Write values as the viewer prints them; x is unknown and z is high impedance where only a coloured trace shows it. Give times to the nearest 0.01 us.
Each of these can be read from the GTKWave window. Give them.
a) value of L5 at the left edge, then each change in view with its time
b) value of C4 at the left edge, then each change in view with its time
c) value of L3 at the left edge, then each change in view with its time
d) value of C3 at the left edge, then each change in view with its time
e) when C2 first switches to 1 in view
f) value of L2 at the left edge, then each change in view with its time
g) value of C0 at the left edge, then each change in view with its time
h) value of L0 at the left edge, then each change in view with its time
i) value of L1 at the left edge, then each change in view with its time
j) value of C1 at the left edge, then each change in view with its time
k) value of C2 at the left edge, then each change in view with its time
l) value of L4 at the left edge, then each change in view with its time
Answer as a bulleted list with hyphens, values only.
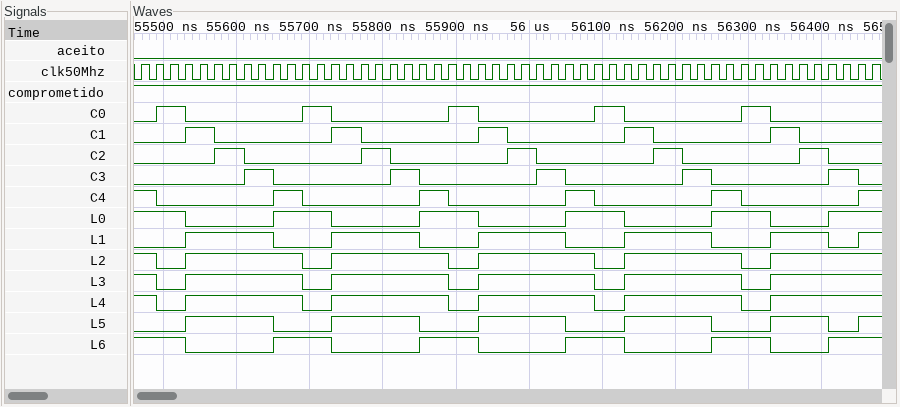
- 0, 1 at 55.53 us, 0 at 55.65 us, 1 at 55.73 us, 0 at 55.85 us, 1 at 55.93 us, 0 at 56.05 us, 1 at 56.13 us, 0 at 56.25 us, 1 at 56.33 us, 0 at 56.41 us, 1 at 56.45 us
- 1, 0 at 55.49 us, 1 at 55.65 us, 0 at 55.69 us, 1 at 55.85 us, 0 at 55.89 us, 1 at 56.05 us, 0 at 56.09 us, 1 at 56.25 us, 0 at 56.29 us, 1 at 56.45 us
- 1, 0 at 55.49 us, 1 at 55.53 us, 0 at 55.69 us, 1 at 55.73 us, 0 at 55.89 us, 1 at 55.93 us, 0 at 56.09 us, 1 at 56.13 us, 0 at 56.29 us, 1 at 56.33 us
- 0, 1 at 55.61 us, 0 at 55.65 us, 1 at 55.81 us, 0 at 55.85 us, 1 at 56.01 us, 0 at 56.05 us, 1 at 56.21 us, 0 at 56.25 us, 1 at 56.41 us, 0 at 56.45 us
- 55.57 us
- 1, 0 at 55.49 us, 1 at 55.53 us, 0 at 55.69 us, 1 at 55.73 us, 0 at 55.89 us, 1 at 55.93 us, 0 at 56.09 us, 1 at 56.13 us, 0 at 56.29 us, 1 at 56.33 us
- 0, 1 at 55.49 us, 0 at 55.53 us, 1 at 55.69 us, 0 at 55.73 us, 1 at 55.89 us, 0 at 55.93 us, 1 at 56.09 us, 0 at 56.13 us, 1 at 56.29 us, 0 at 56.33 us
- 1, 0 at 55.53 us, 1 at 55.65 us, 0 at 55.73 us, 1 at 55.85 us, 0 at 55.93 us, 1 at 56.05 us, 0 at 56.13 us, 1 at 56.25 us, 0 at 56.33 us, 1 at 56.41 us
- 0, 1 at 55.53 us, 0 at 55.65 us, 1 at 55.73 us, 0 at 55.85 us, 1 at 55.93 us, 0 at 56.05 us, 1 at 56.13 us, 0 at 56.25 us, 1 at 56.33 us, 0 at 56.41 us, 1 at 56.45 us
- 0, 1 at 55.53 us, 0 at 55.57 us, 1 at 55.73 us, 0 at 55.77 us, 1 at 55.93 us, 0 at 55.97 us, 1 at 56.13 us, 0 at 56.17 us, 1 at 56.33 us, 0 at 56.37 us
- 0, 1 at 55.57 us, 0 at 55.61 us, 1 at 55.77 us, 0 at 55.81 us, 1 at 55.97 us, 0 at 56.01 us, 1 at 56.17 us, 0 at 56.21 us, 1 at 56.37 us, 0 at 56.41 us
- 1, 0 at 55.49 us, 1 at 55.53 us, 0 at 55.69 us, 1 at 55.73 us, 0 at 55.89 us, 1 at 55.93 us, 0 at 56.09 us, 1 at 56.13 us, 0 at 56.29 us, 1 at 56.33 us
